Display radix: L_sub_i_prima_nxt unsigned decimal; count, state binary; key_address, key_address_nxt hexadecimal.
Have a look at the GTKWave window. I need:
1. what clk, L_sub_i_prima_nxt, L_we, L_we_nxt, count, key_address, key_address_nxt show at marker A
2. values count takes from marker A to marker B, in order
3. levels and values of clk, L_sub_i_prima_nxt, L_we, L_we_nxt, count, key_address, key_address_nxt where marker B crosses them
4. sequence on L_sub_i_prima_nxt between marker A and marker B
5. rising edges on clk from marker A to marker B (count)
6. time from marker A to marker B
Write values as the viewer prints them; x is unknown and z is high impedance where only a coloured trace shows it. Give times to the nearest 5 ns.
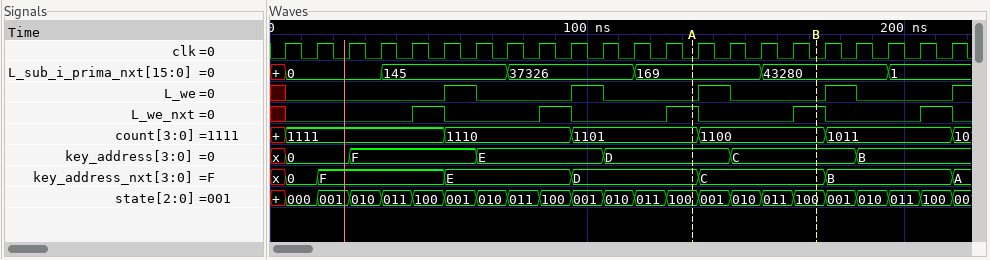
clk=0, L_sub_i_prima_nxt=169, L_we=0, L_we_nxt=1, count=1101, key_address=D, key_address_nxt=D
1101, 1100
clk=0, L_sub_i_prima_nxt=43280, L_we=0, L_we_nxt=1, count=1100, key_address=C, key_address_nxt=C
169, 43280
4
40 ns
